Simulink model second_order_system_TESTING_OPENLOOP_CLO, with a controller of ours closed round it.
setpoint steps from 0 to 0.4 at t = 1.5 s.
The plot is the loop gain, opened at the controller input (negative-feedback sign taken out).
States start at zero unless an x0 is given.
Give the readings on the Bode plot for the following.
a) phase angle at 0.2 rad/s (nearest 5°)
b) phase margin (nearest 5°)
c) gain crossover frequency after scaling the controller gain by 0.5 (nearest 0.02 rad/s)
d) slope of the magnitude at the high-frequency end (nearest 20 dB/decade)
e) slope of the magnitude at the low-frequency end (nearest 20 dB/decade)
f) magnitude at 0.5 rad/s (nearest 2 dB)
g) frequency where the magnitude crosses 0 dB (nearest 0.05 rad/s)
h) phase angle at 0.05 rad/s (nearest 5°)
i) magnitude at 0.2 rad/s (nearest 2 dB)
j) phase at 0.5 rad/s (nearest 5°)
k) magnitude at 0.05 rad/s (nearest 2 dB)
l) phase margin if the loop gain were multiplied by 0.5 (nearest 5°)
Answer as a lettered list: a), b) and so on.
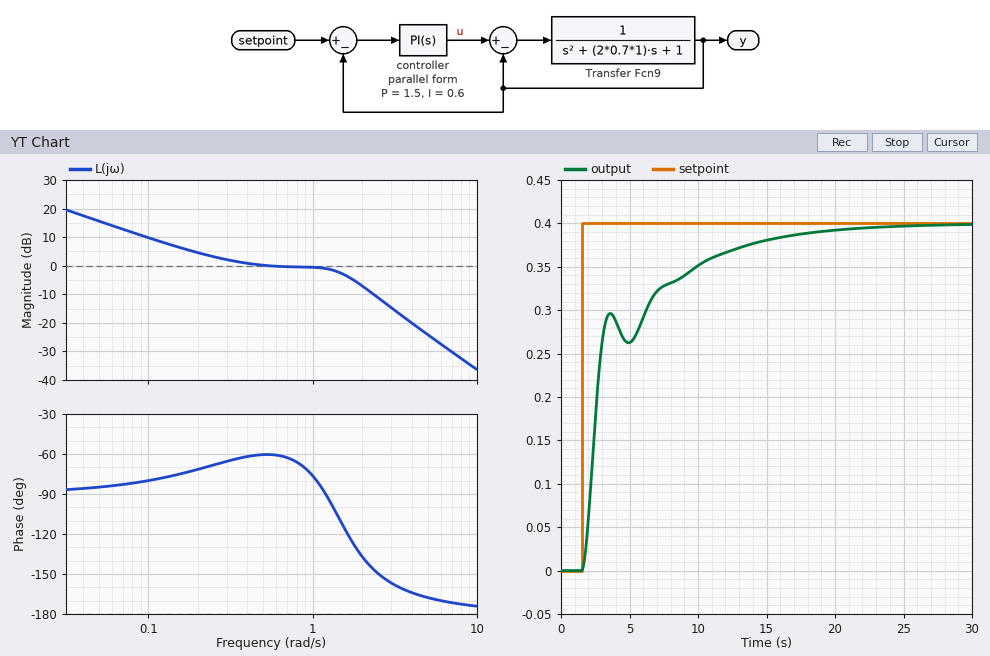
a) -70°
b) 120°
c) 0.16 rad/s
d) -40 dB/decade
e) -20 dB/decade
f) 0 dB
g) 0.55 rad/s
h) -85°
i) 4 dB
j) -60°
k) 16 dB
l) 105°
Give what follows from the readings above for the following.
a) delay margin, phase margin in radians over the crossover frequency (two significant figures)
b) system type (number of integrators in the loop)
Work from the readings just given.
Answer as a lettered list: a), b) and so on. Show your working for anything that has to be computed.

a) 120 × π / 180 / 0.55 = 3.8 s
b) 1
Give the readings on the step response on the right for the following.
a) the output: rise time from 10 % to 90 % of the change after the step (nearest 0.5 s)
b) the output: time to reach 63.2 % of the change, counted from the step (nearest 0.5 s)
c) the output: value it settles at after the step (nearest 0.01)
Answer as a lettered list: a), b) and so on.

a) 9.0 s
b) 1.5 s
c) 0.40
